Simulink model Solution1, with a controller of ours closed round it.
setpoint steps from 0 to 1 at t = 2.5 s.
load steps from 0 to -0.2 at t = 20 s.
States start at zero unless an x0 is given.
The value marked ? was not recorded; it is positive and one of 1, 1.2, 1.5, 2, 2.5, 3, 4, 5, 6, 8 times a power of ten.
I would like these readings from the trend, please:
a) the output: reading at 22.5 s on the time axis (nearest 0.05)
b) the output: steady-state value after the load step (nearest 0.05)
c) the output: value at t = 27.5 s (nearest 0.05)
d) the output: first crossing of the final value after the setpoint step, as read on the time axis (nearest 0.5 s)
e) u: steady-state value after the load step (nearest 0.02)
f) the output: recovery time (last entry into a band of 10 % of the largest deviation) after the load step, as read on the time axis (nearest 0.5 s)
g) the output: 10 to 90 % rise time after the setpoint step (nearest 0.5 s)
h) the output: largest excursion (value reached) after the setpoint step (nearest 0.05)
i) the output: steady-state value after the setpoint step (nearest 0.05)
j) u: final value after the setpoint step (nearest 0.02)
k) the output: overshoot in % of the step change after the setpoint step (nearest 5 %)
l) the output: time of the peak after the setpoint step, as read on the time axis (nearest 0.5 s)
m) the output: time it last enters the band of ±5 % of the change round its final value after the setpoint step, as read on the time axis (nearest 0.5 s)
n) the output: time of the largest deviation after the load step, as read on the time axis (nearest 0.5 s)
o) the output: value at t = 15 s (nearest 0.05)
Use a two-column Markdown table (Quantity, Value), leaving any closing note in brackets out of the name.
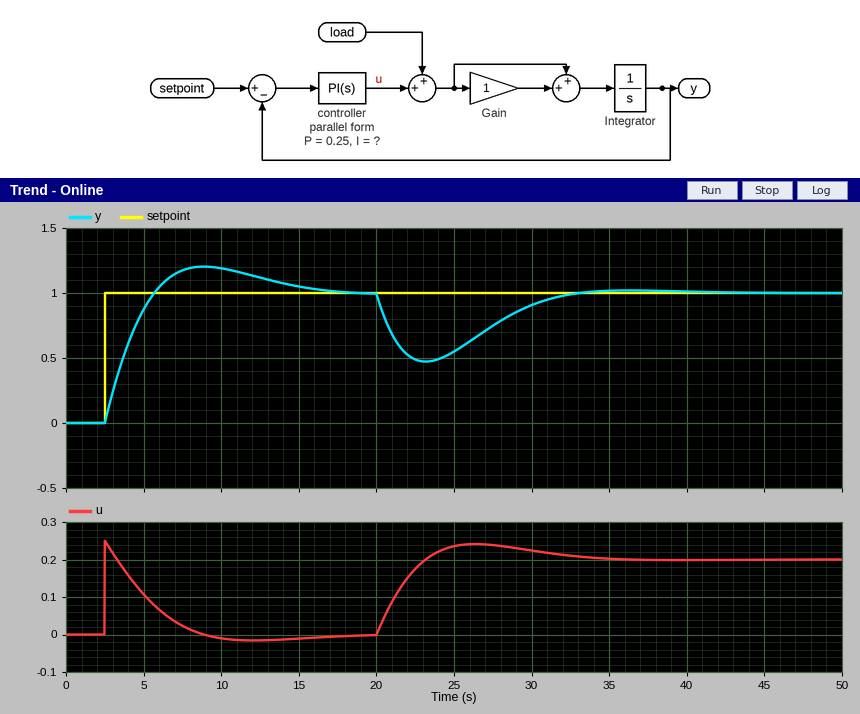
| Quantity | Value |
|---|---|
| the output: reading at 22.5 s on the time axis | 0.50 |
| the output: steady-state value after the load step | 1.00 |
| the output: value at t = 27.5 s | 0.75 |
| the output: first crossing of the final value after the setpoint step, as read on the time axis | 5.5 s |
| u: steady-state value after the load step | 0.20 |
| the output: recovery time (last entry into a band of 10 % of the largest deviation) after the load step, as read on the time axis | 31.0 s |
| the output: 10 to 90 % rise time after the setpoint step | 2.5 s |
| the output: largest excursion (value reached) after the setpoint step | 1.20 |
| the output: steady-state value after the setpoint step | 1.00 |
| u: final value after the setpoint step | 0.00 |
| the output: overshoot in % of the step change after the setpoint step | 20 % |
| the output: time of the peak after the setpoint step, as read on the time axis | 9.0 s |
| the output: time it last enters the band of ±5 % of the change round its final value after the setpoint step, as read on the time axis | 15.0 s |
| the output: time of the largest deviation after the load step, as read on the time axis | 23.0 s |
| the output: value at t = 15 s | 1.05 |
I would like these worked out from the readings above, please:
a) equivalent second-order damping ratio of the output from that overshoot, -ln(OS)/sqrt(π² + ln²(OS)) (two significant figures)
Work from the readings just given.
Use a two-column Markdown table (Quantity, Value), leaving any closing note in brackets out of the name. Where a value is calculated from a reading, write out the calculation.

| Quantity | Value |
|---|---|
| equivalent second-order damping ratio of the output from that overshoot, -ln(OS)/sqrt(π² + ln²(OS)) | ln(0.2) = -1.609; 1.609 / sqrt(9.870 + 2.590) = 0.46 |
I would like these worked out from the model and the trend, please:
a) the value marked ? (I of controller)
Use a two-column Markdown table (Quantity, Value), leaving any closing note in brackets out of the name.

| Quantity | Value |
|---|---|
| the value marked ? | 0.06 |
